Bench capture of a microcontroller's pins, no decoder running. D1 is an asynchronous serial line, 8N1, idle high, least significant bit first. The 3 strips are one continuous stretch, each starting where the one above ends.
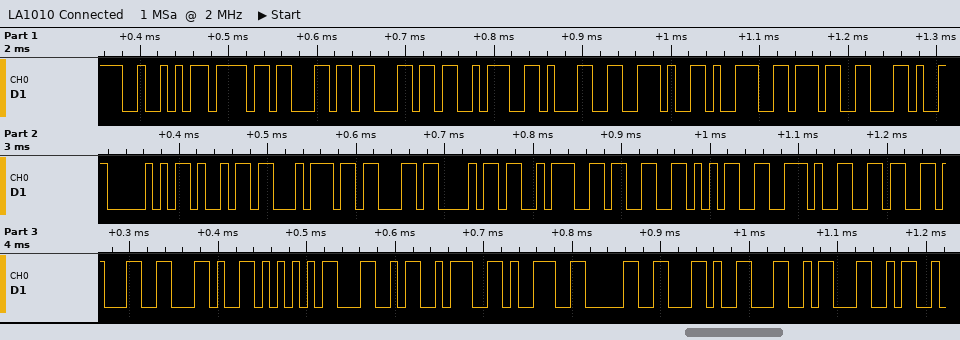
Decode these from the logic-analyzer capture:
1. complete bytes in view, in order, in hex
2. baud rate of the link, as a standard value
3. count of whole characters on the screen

0x52 0x6F 0x6C 0x6C 0x3A 0x31 0x2E 0x39 0x37 0x2C 0x50 0x69 0x74 0x63 0x68 0x3A 0x33 0x35 0x2E 0x36 0x31 0x2C 0x55 0x4C 0x3A 0x39 0x30 0x2C 0x4C 0x4C
115200 baud
30
